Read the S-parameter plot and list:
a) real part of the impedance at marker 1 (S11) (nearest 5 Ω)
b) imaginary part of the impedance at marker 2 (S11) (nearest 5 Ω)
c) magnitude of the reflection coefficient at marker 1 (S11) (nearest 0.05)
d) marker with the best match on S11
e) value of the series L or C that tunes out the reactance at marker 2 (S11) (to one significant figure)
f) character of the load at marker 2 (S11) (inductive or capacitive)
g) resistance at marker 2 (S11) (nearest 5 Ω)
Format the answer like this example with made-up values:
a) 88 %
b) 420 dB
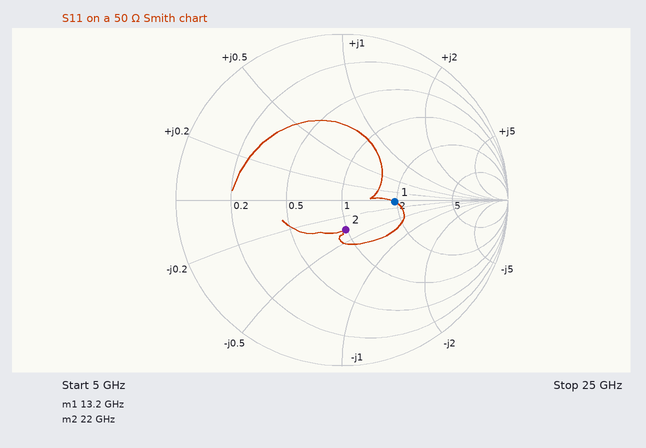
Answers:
a) 95 Ω
b) -20 Ω
c) 0.30
d) marker 2
e) 100 pH
f) capacitive
g) 50 Ω
